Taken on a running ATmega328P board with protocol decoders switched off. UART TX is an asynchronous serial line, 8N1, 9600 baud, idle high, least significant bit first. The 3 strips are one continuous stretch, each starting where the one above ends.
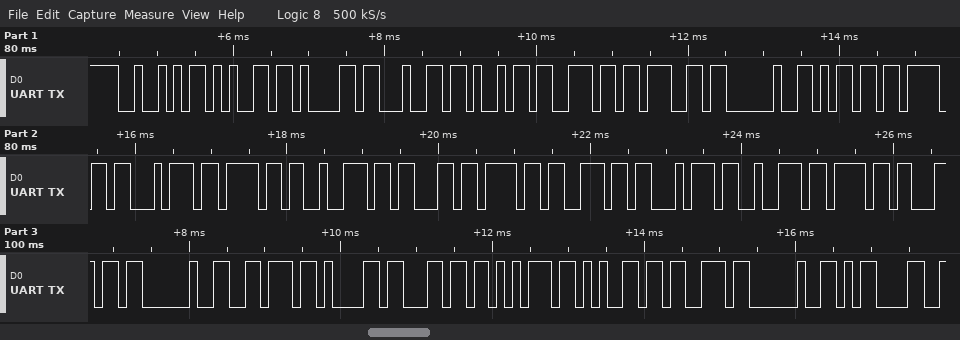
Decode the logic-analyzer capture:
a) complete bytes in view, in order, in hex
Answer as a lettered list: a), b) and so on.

a) 0x52 0x65 0x61 0x64 0x69 0x6E 0x67 0x20 0x6D 0x6F 0x74 0x6F 0x72 0x63 0x6F 0x6E 0x74 0x72 0x6F 0x6C 0x20 0x76 0x61 0x6C 0x75 0x65 0x73 0x20 0x0D
